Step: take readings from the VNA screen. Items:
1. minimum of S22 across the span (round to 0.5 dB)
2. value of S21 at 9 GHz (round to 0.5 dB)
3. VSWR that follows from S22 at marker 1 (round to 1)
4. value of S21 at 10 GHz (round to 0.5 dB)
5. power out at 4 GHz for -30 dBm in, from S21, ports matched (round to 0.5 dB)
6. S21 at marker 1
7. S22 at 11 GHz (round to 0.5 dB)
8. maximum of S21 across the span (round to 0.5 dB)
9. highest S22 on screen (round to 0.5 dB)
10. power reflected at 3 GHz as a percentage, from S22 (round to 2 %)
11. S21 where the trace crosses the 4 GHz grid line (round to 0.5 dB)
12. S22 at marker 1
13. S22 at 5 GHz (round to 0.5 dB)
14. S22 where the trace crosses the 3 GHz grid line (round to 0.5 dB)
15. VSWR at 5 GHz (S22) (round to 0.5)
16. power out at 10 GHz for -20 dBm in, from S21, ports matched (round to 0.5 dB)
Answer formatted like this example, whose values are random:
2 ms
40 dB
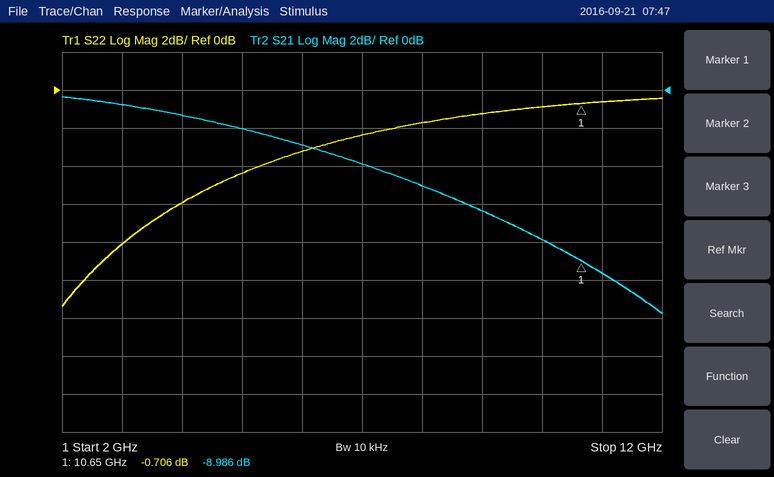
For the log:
-11.5 dB
-6.5 dB
25
-8.0 dB
-31.5 dBm
-8.986 dB
-0.5 dB
-0.5 dB
-0.5 dB
16 %
-1.5 dB
-0.706 dB
-4.5 dB
-8.0 dB
4.0
-28.0 dBm
